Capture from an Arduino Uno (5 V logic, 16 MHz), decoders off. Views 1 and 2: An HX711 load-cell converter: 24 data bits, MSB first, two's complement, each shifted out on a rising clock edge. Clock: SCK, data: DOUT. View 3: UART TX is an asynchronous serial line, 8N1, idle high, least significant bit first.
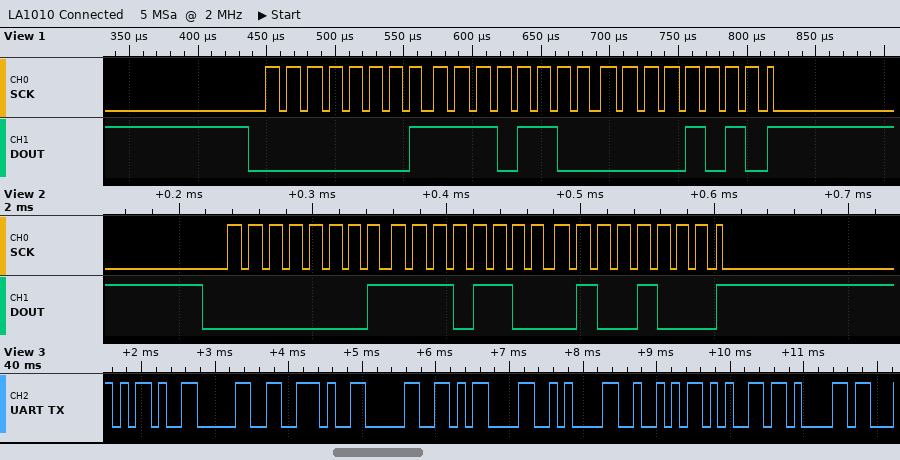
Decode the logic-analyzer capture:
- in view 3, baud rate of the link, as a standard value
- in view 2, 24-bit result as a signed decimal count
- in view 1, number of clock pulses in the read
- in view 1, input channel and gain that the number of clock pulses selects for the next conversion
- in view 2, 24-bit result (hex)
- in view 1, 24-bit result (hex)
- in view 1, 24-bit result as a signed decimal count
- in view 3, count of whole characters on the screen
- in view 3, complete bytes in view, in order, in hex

9600 baud
126024
25
channel A, gain 128
0x01EC48
0x01EC0A
125962
9
0x2D 0x30 0x2E 0x30 0x0D 0x0A 0x52 0x65 0x61
